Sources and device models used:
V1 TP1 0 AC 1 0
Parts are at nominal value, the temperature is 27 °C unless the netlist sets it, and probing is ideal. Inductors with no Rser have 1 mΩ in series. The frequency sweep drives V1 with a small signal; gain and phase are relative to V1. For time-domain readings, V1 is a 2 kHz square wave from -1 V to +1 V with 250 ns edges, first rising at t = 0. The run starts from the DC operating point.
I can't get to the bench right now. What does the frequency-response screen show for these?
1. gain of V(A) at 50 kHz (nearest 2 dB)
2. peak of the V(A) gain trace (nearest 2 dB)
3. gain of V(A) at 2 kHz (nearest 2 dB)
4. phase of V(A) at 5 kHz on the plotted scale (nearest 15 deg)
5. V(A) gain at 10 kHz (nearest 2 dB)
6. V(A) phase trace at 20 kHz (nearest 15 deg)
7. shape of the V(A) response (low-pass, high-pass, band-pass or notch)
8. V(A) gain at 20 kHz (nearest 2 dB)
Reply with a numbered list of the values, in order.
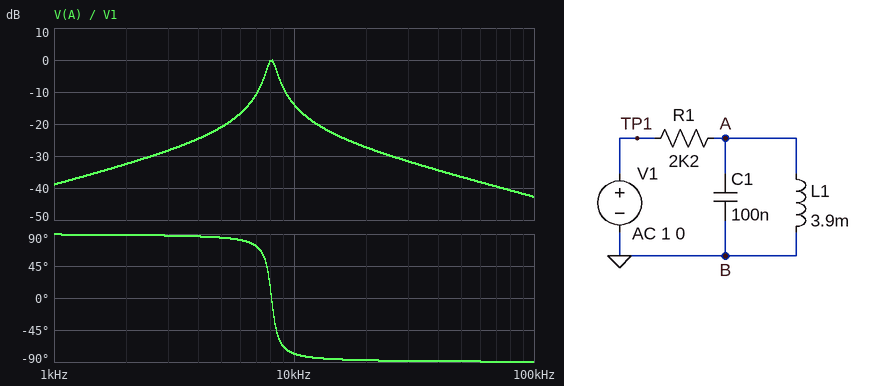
1. -36 dB
2. 0 dB
3. -32 dB
4. 90 deg
5. -14 dB
6. -90 deg
7. band-pass
8. -28 dB
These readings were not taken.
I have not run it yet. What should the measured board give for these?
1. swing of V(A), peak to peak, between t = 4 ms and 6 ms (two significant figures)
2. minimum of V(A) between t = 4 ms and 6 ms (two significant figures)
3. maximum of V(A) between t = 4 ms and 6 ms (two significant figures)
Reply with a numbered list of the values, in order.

1. 210 mV
2. -110 mV
3. 110 mV
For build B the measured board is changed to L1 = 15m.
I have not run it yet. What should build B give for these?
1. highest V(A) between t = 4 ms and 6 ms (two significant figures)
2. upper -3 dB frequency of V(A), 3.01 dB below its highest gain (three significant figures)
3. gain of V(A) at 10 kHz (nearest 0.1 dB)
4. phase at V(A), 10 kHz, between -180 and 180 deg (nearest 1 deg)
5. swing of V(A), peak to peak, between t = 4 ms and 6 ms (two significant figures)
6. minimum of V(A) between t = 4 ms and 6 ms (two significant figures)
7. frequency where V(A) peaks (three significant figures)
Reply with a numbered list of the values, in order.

1. 200 mV
2. 4.49 kHz
3. -21.2 dB
4. -85 deg
5. 390 mV
6. -200 mV
7. 4.11 kHz
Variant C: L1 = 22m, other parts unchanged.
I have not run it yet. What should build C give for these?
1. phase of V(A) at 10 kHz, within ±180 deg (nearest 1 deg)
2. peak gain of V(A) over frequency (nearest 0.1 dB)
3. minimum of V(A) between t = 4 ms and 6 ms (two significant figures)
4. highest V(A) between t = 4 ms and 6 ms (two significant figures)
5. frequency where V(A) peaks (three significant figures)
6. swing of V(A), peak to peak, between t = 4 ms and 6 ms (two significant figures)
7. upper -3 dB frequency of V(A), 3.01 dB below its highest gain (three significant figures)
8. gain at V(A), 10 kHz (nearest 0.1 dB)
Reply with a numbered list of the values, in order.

1. -85 deg
2. 0 dB
3. -270 mV
4. 270 mV
5. 3.39 kHz
6. 540 mV
7. 3.77 kHz
8. -21.8 dB
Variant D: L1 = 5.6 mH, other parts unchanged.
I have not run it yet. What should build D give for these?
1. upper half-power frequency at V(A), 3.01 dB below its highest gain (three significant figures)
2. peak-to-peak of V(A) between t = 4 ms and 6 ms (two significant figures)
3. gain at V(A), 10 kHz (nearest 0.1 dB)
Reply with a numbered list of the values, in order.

1. 7.10 kHz
2. 450 mV
3. -17.7 dB
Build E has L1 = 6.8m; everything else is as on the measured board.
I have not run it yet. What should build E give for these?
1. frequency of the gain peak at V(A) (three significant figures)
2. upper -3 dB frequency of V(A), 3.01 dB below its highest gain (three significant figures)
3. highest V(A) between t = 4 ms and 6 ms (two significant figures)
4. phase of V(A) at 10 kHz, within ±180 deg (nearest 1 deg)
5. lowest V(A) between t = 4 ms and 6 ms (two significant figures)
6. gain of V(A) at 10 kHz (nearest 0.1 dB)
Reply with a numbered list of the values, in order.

1. 6.10 kHz
2. 6.48 kHz
3. 490 mV
4. -83 deg
5. -490 mV
6. -18.8 dB
